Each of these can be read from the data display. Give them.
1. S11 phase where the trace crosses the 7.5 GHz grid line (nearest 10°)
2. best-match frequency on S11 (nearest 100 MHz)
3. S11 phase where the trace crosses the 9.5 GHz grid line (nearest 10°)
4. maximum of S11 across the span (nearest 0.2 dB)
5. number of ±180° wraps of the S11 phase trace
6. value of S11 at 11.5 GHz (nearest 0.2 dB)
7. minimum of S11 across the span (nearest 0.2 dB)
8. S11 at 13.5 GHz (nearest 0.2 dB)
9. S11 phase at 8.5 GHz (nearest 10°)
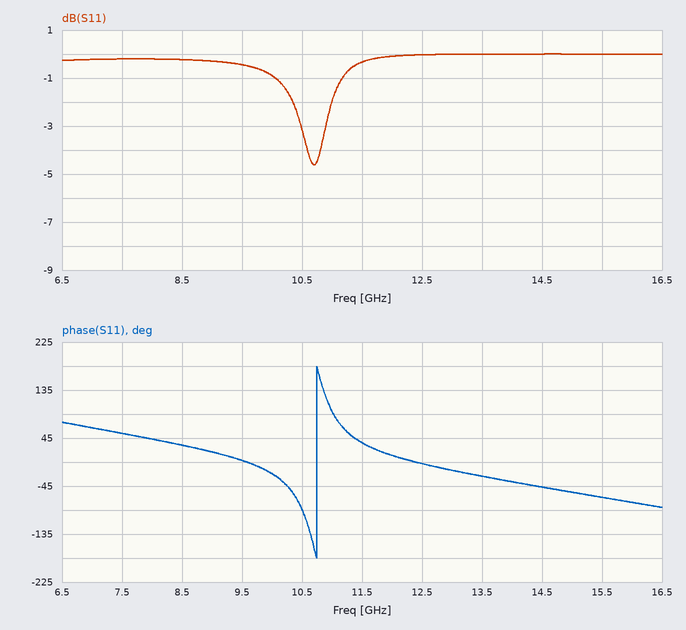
50°
10.7 GHz
0°
0.0 dB
1
-0.4 dB
-4.6 dB
0.0 dB
30°
